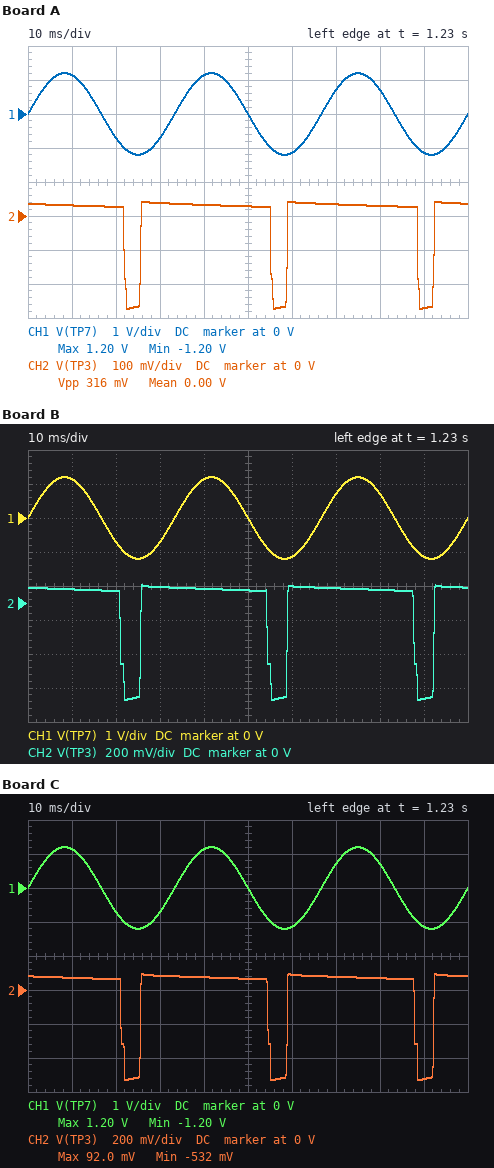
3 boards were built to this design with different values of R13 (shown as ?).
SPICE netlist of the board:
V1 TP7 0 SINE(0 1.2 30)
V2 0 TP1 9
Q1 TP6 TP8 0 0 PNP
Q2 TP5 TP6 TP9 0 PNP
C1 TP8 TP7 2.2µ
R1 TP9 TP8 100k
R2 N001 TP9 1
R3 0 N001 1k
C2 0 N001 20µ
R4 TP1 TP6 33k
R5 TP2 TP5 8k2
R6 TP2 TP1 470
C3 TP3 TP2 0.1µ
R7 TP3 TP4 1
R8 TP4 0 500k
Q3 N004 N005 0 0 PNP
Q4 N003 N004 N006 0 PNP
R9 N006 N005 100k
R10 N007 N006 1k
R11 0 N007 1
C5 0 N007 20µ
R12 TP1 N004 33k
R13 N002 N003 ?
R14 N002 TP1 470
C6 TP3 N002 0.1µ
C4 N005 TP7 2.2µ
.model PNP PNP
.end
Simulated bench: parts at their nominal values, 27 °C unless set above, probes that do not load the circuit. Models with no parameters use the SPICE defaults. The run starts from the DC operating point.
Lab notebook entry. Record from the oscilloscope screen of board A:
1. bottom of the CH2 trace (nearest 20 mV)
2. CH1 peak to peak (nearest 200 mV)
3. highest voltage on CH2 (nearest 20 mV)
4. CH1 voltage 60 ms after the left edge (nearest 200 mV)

-280 mV
2.4 V
40 mV
-1.2 V
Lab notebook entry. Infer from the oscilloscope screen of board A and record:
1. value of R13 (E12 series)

22 kΩ
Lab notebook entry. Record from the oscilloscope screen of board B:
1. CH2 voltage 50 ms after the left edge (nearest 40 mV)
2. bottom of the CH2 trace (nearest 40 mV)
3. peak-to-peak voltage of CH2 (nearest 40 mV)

80 mV
-560 mV
680 mV
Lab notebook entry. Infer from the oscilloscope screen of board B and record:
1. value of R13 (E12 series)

3.3 kΩ
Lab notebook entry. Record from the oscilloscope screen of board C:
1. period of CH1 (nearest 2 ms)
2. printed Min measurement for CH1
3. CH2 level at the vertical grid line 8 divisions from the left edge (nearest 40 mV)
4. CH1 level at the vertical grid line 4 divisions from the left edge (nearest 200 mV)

34 ms
-1.20 V
80 mV
1.2 V
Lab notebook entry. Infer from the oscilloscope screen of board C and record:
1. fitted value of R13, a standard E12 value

3.9 kΩ
